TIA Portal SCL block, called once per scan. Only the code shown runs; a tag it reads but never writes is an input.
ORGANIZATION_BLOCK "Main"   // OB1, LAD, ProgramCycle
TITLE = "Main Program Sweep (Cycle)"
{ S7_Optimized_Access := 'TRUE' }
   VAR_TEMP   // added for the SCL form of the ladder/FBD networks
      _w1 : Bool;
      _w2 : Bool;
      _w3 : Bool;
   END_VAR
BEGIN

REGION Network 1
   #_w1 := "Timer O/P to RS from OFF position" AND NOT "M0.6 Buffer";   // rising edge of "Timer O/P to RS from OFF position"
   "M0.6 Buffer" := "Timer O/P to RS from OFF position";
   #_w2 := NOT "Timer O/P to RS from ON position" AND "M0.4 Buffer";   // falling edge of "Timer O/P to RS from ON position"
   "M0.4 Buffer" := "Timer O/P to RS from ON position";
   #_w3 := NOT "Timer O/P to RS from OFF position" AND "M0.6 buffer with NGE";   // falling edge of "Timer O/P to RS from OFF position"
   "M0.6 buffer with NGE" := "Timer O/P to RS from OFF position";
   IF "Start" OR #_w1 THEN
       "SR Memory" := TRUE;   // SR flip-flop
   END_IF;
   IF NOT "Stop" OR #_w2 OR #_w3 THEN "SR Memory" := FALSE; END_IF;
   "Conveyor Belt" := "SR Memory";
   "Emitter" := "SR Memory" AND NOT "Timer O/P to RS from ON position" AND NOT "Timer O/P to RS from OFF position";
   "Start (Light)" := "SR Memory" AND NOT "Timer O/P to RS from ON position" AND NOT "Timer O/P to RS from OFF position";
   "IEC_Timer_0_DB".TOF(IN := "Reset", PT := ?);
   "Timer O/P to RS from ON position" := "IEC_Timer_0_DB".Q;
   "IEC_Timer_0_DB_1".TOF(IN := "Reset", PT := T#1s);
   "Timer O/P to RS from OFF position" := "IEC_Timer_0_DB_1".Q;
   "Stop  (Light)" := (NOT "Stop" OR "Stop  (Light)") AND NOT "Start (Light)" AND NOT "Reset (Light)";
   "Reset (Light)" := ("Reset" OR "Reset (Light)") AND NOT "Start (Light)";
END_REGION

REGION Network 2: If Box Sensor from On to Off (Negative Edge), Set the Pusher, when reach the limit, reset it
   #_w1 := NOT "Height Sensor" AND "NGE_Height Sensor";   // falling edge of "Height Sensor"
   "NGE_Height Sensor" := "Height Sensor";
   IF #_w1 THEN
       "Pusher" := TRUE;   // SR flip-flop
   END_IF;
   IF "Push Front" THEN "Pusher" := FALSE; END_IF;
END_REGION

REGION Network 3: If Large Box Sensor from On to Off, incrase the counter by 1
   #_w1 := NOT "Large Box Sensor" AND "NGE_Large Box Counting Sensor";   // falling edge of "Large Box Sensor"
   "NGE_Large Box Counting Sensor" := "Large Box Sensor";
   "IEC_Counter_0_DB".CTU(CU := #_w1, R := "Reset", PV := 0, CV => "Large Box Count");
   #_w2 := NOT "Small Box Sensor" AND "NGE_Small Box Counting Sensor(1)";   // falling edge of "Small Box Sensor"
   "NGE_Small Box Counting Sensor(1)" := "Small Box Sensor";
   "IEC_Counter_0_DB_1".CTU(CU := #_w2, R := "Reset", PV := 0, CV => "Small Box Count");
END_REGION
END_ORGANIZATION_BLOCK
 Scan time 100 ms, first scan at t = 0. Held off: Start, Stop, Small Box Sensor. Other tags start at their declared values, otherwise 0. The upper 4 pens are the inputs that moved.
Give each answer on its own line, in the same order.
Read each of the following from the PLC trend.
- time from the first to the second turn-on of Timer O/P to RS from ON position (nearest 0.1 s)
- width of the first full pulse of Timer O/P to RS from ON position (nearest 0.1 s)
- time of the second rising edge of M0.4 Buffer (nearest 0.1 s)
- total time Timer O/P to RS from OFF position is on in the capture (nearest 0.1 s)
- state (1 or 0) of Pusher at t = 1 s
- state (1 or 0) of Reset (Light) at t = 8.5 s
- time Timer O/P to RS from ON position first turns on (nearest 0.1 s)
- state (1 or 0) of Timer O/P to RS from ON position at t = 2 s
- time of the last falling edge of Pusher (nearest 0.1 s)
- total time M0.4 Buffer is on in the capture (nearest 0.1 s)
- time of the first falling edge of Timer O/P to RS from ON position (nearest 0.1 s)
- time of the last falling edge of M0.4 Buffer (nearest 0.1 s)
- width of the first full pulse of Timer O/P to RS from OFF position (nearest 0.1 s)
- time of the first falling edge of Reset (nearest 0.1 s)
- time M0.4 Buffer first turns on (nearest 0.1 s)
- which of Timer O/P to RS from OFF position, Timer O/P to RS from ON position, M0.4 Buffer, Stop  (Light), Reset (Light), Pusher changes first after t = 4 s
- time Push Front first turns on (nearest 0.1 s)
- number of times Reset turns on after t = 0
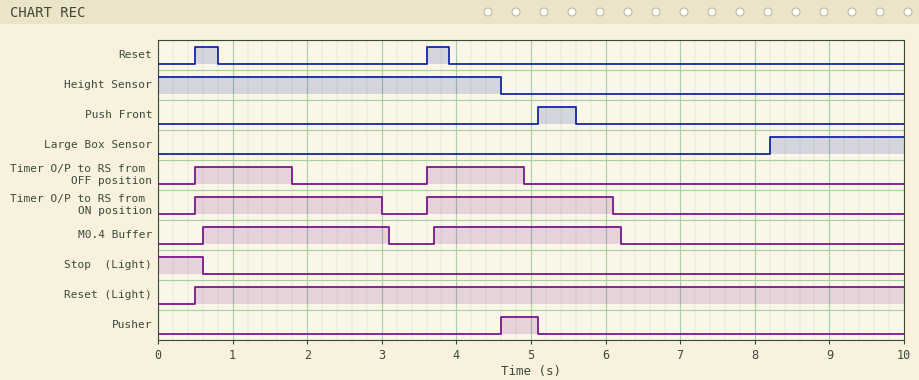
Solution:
3.1 s
2.5 s
3.7 s
2.6 s
0
1
0.5 s
1
5.1 s
5.0 s
3.0 s
6.2 s
1.3 s
0.8 s
0.6 s
Pusher
5.1 s
2
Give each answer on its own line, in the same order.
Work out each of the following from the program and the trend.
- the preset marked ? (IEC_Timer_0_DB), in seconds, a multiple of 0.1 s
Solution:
2.2 s
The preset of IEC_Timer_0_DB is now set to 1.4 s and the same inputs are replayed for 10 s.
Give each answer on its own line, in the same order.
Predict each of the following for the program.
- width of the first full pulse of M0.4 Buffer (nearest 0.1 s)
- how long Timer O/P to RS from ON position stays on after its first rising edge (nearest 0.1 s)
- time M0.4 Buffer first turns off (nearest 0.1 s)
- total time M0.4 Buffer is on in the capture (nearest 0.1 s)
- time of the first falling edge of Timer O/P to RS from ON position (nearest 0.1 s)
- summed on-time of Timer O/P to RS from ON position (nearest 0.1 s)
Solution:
1.7 s
1.7 s
2.3 s
3.4 s
2.2 s
3.4 s
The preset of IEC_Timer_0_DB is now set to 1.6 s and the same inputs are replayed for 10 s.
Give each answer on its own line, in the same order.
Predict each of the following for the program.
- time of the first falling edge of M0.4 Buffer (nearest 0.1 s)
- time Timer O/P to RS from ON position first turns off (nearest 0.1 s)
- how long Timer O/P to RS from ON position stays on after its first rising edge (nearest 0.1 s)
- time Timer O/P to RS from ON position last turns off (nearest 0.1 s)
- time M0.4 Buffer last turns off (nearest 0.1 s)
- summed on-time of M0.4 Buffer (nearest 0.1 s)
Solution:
2.5 s
2.4 s
1.9 s
5.5 s
5.6 s
3.8 s
